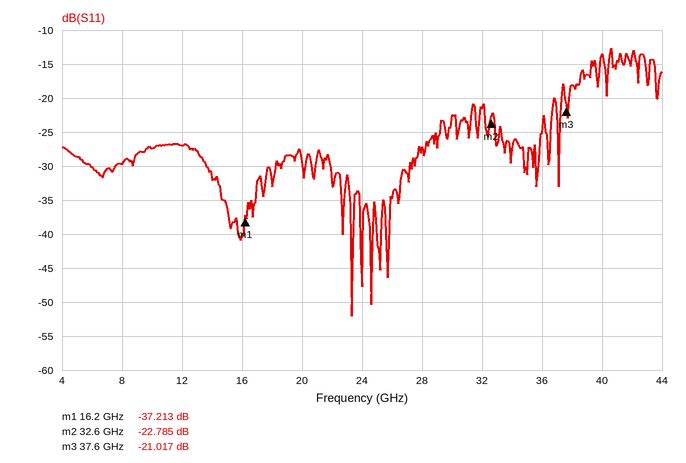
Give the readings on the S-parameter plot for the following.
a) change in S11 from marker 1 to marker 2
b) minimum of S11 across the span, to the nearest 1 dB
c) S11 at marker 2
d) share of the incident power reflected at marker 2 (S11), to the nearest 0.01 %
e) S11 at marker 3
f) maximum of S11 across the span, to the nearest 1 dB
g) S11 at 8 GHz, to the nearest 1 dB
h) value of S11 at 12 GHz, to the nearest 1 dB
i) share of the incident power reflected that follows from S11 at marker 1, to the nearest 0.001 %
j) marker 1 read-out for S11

14.428 dB
-52 dB
-22.785 dB
0.53 %
-21.017 dB
-13 dB
-30 dB
-27 dB
0.019 %
-37.213 dB
